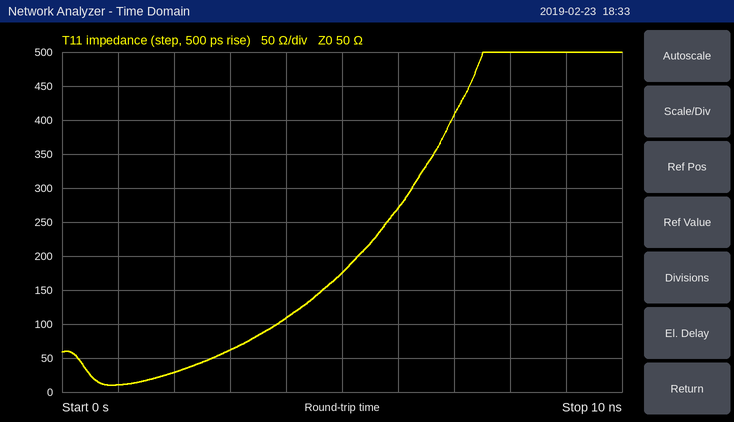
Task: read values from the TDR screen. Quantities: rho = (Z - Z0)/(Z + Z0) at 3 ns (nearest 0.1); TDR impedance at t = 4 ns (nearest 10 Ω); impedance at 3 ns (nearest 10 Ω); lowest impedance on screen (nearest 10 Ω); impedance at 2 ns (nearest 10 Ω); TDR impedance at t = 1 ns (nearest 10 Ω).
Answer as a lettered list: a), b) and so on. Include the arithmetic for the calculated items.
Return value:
a) (60 − 50)/(60 + 50) ≈ +0.1
b) 110 Ω
c) 60 Ω
d) 10 Ω
e) 30 Ω
f) 10 Ω
